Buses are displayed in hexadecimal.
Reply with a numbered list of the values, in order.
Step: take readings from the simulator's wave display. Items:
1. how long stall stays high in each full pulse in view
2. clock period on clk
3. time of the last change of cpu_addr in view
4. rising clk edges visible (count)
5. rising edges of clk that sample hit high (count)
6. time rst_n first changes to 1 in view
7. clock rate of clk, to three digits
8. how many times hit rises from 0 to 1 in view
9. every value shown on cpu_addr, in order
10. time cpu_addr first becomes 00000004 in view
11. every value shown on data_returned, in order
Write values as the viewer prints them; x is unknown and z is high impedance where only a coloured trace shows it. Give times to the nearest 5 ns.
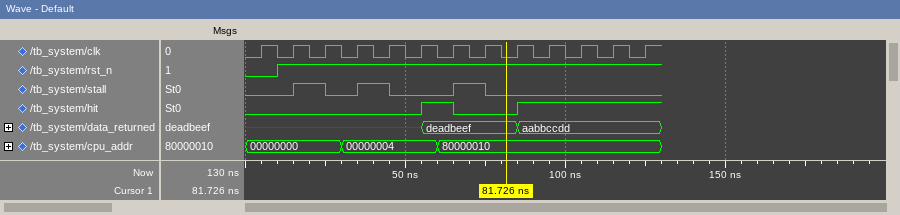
1. 10 ns, 10 ns, 10 ns
2. 10 ns
3. 60 ns
4. 13
5. 5
6. 10 ns
7. 100 MHz
8. 2
9. 00000000, 00000004, 80000010
10. 30 ns
11. x, deadbeef, aabbccdd
